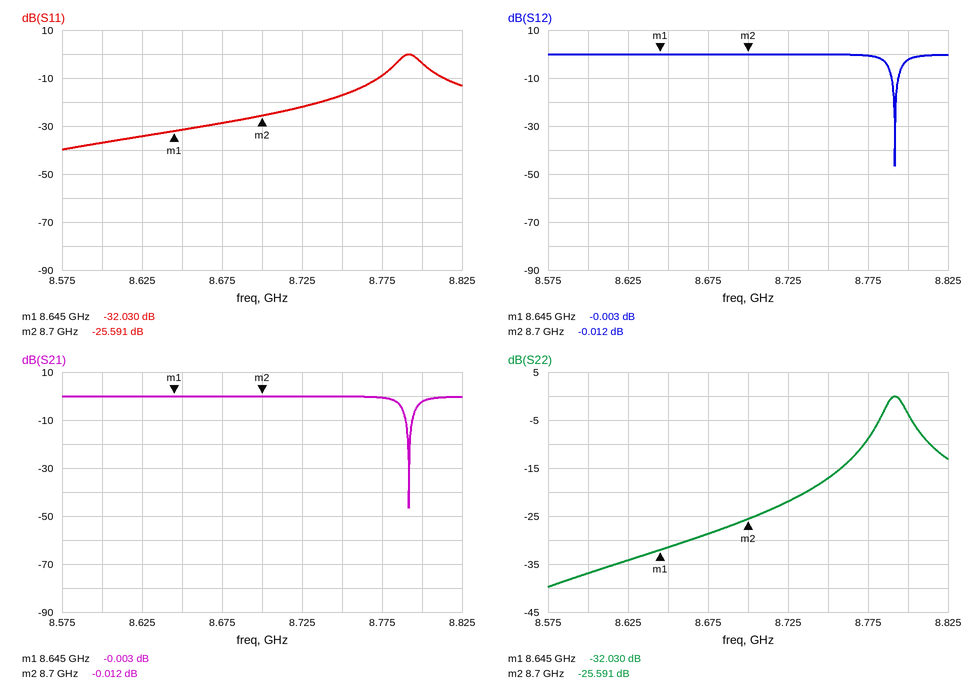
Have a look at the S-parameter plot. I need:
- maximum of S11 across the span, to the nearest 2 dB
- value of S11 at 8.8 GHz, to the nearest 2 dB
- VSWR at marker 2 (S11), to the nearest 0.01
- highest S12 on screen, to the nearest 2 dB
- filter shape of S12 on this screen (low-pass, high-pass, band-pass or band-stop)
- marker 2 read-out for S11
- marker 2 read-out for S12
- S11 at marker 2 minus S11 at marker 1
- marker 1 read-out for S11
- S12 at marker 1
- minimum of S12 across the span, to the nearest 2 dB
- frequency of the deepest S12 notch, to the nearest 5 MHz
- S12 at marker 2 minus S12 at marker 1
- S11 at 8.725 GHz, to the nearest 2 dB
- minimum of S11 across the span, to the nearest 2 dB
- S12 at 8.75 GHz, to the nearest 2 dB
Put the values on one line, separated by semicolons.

0 dB; -4 dB; 1.11; 0 dB; band-stop; -25.591 dB; -0.012 dB; 6.439 dB; -32.030 dB; -0.003 dB; -46 dB; 8.790 GHz; -0.009 dB; -22 dB; -40 dB; 0 dB
